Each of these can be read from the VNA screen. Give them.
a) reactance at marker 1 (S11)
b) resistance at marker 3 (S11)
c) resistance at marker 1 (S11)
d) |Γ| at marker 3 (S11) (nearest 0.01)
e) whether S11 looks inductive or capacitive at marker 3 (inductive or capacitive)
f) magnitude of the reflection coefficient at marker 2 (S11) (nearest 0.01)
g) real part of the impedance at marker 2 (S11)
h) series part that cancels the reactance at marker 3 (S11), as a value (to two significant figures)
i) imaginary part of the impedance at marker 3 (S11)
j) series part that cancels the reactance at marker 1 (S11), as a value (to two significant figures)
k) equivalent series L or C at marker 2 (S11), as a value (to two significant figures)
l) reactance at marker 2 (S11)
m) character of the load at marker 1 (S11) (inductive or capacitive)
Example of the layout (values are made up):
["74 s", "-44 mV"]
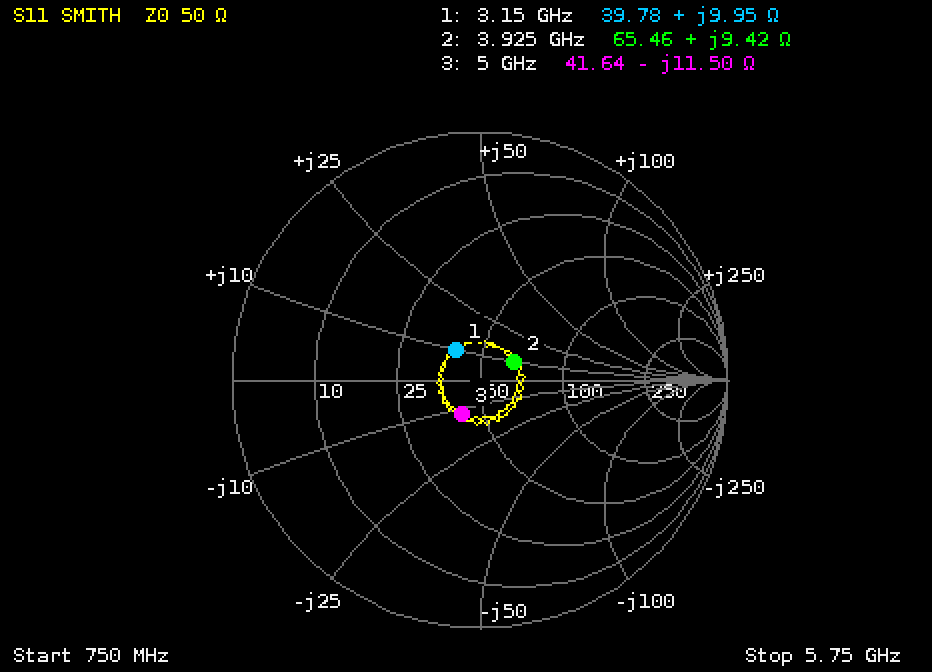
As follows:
["+9.95 Ω", "41.64 Ω", "39.78 Ω", "0.15", "capacitive", "0.16", "65.46 Ω", "370 pH", "-11.50 Ω", "5.1 pF", "380 pH", "+9.42 Ω", "inductive"]
